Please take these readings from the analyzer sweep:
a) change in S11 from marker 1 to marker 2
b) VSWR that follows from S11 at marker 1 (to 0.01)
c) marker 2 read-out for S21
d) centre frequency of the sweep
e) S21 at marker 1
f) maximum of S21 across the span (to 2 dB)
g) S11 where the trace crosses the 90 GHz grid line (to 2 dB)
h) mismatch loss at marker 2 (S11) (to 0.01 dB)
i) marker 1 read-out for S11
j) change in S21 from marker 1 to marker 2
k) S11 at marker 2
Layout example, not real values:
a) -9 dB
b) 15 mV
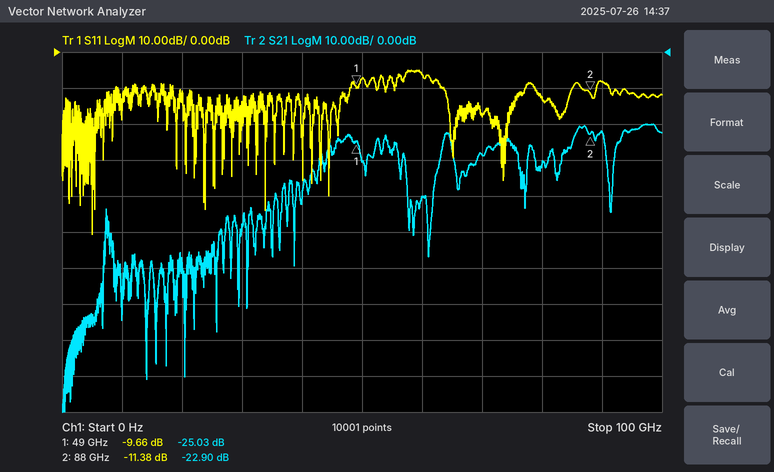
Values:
a) -1.72 dB
b) 1.98
c) -22.90 dB
d) 50 GHz
e) -25.03 dB
f) -20 dB
g) -8 dB
h) 0.33 dB
i) -9.66 dB
j) 2.13 dB
k) -11.38 dB
